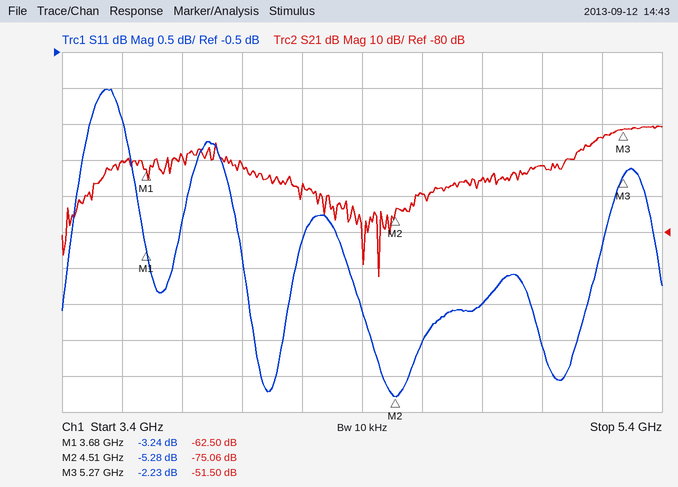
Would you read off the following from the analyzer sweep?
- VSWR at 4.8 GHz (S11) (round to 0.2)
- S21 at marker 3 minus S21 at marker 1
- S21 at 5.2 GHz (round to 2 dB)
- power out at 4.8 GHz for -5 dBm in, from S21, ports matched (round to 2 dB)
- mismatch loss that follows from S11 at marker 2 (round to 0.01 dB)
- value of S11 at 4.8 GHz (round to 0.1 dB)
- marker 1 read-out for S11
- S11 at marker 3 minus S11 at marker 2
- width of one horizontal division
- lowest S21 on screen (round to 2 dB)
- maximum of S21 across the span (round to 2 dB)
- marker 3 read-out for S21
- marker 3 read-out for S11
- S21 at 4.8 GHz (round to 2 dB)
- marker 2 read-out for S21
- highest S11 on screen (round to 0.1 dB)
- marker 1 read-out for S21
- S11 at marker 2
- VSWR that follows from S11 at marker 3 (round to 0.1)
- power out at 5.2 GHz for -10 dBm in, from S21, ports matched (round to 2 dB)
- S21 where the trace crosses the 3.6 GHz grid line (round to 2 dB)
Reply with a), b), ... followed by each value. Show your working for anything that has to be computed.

a) |Γ| = 10^(-4/20) = 0.6310; VSWR = (1 + 0.6310)/(1 − 0.6310) ≈ 4.4
b) -51.5 − (-62.5) = 11.00 dB
c) -54 dB
d) -5 dBm + (-66 dB) = -70 dBm
e) −10 log10(1 − 10^(-5.28/10)) ≈ 1.53 dB
f) -4.0 dB
g) -3.24 dB
h) -2.23 − (-5.28) = 3.05 dB
i) 200 MHz
j) -92 dB
k) -50 dB
l) -51.50 dB
m) -2.23 dB
n) -66 dB
o) -75.06 dB
p) -1.0 dB
q) -62.50 dB
r) -5.28 dB
s) (1 + 0.7736)/(1 − 0.7736) ≈ 7.8
t) -10 dBm + (-54 dB) = -64 dBm
u) -60 dB
